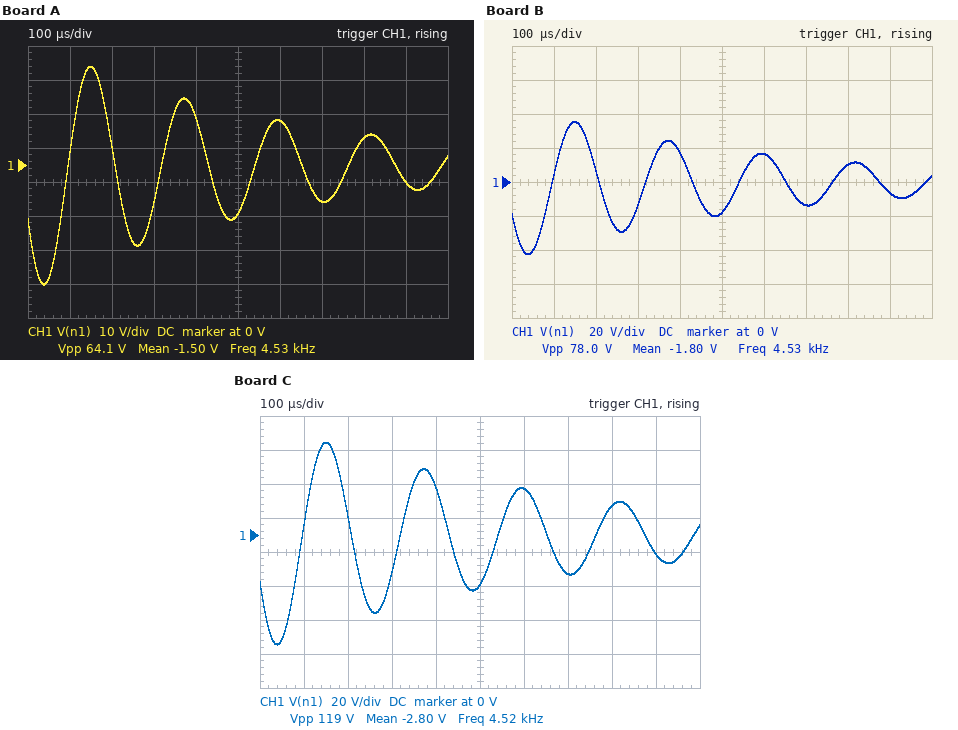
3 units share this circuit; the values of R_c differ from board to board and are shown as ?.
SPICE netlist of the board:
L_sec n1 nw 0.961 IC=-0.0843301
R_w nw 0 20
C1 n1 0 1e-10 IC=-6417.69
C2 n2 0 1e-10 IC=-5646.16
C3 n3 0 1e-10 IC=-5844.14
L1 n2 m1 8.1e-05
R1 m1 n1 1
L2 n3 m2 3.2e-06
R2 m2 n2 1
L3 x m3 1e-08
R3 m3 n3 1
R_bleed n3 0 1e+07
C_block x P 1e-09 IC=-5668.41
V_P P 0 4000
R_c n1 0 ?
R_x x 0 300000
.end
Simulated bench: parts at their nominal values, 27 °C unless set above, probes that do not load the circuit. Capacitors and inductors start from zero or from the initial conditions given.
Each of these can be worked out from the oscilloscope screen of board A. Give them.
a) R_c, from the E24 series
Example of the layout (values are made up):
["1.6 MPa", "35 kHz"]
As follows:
["910 kΩ"]
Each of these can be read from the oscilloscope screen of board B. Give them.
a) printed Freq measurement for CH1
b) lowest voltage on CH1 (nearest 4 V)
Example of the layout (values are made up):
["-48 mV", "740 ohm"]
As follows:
["4.53 kHz", "-44 V"]
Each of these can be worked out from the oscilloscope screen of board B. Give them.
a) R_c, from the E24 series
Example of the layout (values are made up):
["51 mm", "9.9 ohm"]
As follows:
["1.1 MΩ"]
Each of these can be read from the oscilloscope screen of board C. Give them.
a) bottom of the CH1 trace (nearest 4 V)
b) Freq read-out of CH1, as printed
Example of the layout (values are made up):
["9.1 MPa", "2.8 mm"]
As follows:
["-64 V", "4.52 kHz"]
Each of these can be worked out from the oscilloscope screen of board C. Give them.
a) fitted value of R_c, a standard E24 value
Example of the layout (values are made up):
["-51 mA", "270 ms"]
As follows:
["2 MΩ"]
